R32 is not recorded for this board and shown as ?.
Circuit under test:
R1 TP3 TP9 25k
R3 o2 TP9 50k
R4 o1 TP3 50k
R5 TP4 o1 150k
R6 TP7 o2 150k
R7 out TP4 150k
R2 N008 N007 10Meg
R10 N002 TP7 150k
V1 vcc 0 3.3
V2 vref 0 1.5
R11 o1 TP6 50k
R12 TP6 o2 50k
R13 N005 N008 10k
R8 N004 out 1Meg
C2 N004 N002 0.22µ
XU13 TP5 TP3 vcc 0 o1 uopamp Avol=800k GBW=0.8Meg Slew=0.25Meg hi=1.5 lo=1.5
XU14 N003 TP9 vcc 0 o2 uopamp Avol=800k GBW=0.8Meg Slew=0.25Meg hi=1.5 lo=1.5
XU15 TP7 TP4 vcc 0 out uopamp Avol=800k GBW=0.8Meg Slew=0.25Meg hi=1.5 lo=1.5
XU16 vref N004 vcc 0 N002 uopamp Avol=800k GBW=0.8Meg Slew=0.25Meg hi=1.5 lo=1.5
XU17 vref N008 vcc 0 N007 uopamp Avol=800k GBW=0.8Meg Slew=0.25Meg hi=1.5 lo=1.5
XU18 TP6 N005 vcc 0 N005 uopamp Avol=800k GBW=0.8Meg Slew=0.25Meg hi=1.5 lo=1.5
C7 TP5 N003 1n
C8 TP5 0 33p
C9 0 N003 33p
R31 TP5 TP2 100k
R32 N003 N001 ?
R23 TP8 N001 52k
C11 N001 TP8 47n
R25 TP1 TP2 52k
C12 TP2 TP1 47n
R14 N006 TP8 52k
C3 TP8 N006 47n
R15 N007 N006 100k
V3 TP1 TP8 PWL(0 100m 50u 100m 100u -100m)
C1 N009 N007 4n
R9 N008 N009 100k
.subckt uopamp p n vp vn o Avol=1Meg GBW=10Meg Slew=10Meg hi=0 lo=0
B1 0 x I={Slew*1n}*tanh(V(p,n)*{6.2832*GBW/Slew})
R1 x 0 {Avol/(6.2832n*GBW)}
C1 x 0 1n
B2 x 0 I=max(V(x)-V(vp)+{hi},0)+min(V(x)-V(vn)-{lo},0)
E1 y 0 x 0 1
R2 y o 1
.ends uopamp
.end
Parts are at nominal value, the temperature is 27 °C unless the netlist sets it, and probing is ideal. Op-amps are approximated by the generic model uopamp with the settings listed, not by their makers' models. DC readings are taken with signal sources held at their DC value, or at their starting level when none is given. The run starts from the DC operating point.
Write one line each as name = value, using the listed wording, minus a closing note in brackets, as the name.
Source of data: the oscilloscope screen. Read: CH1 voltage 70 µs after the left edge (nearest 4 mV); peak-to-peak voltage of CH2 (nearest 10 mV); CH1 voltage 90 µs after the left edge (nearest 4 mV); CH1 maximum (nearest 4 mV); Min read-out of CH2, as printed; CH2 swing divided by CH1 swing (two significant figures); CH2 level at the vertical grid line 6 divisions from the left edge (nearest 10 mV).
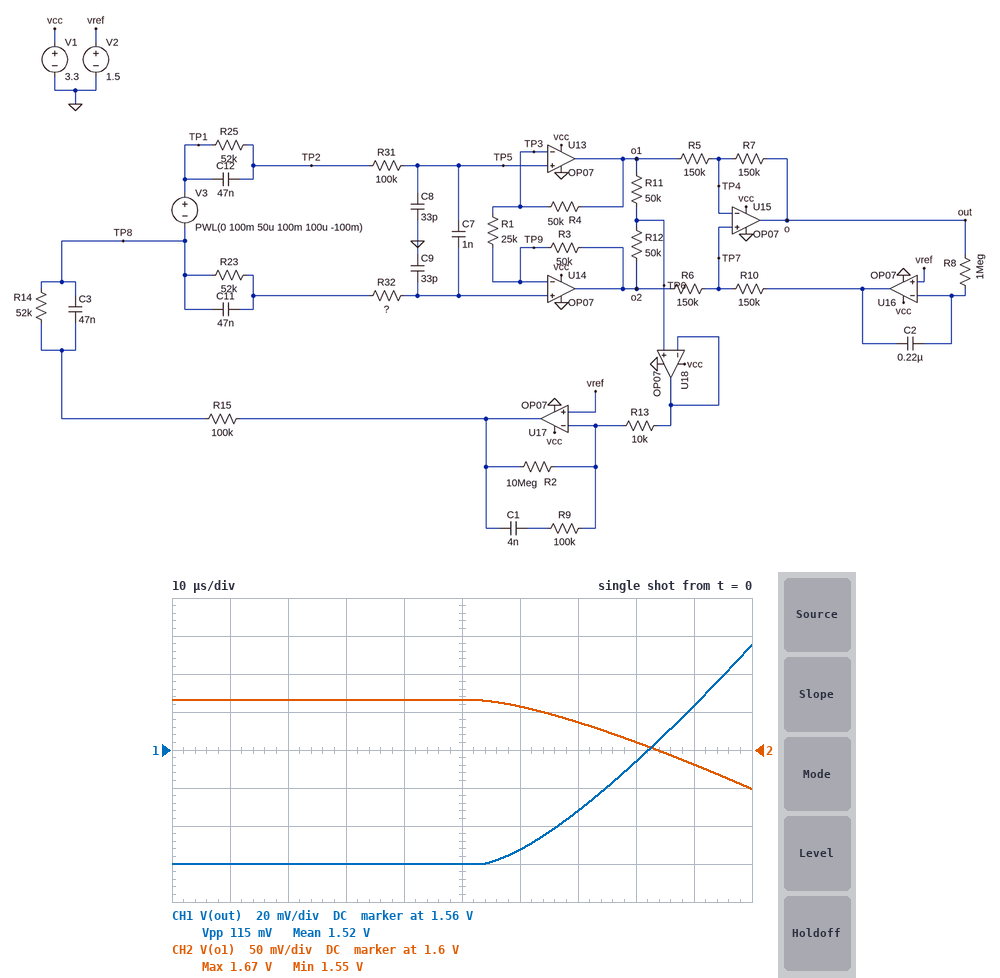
CH1 voltage 70 µs after the left edge = 1.528 V
peak-to-peak voltage of CH2 = 120 mV
CH1 voltage 90 µs after the left edge = 1.584 V
CH1 maximum = 1.616 V
Min read-out of CH2, as printed = 1.55 V
CH2 swing divided by CH1 swing = 1.0
CH2 level at the vertical grid line 6 divisions from the left edge = 1.66 V
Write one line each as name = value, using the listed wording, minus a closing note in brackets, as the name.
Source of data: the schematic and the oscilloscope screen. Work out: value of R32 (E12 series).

value of R32 = 47 kΩ
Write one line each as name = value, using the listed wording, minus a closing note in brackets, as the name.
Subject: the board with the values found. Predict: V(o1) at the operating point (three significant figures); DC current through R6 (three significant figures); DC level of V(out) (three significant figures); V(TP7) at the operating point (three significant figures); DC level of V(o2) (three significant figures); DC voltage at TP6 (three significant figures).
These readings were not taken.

V(o1) at the operating point = 1.67 V
DC current through R6 = 553 nA
DC level of V(out) = 1.50 V
V(TP7) at the operating point = 1.58 V
DC level of V(o2) = 1.50 V
DC voltage at TP6 = 1.58 V
